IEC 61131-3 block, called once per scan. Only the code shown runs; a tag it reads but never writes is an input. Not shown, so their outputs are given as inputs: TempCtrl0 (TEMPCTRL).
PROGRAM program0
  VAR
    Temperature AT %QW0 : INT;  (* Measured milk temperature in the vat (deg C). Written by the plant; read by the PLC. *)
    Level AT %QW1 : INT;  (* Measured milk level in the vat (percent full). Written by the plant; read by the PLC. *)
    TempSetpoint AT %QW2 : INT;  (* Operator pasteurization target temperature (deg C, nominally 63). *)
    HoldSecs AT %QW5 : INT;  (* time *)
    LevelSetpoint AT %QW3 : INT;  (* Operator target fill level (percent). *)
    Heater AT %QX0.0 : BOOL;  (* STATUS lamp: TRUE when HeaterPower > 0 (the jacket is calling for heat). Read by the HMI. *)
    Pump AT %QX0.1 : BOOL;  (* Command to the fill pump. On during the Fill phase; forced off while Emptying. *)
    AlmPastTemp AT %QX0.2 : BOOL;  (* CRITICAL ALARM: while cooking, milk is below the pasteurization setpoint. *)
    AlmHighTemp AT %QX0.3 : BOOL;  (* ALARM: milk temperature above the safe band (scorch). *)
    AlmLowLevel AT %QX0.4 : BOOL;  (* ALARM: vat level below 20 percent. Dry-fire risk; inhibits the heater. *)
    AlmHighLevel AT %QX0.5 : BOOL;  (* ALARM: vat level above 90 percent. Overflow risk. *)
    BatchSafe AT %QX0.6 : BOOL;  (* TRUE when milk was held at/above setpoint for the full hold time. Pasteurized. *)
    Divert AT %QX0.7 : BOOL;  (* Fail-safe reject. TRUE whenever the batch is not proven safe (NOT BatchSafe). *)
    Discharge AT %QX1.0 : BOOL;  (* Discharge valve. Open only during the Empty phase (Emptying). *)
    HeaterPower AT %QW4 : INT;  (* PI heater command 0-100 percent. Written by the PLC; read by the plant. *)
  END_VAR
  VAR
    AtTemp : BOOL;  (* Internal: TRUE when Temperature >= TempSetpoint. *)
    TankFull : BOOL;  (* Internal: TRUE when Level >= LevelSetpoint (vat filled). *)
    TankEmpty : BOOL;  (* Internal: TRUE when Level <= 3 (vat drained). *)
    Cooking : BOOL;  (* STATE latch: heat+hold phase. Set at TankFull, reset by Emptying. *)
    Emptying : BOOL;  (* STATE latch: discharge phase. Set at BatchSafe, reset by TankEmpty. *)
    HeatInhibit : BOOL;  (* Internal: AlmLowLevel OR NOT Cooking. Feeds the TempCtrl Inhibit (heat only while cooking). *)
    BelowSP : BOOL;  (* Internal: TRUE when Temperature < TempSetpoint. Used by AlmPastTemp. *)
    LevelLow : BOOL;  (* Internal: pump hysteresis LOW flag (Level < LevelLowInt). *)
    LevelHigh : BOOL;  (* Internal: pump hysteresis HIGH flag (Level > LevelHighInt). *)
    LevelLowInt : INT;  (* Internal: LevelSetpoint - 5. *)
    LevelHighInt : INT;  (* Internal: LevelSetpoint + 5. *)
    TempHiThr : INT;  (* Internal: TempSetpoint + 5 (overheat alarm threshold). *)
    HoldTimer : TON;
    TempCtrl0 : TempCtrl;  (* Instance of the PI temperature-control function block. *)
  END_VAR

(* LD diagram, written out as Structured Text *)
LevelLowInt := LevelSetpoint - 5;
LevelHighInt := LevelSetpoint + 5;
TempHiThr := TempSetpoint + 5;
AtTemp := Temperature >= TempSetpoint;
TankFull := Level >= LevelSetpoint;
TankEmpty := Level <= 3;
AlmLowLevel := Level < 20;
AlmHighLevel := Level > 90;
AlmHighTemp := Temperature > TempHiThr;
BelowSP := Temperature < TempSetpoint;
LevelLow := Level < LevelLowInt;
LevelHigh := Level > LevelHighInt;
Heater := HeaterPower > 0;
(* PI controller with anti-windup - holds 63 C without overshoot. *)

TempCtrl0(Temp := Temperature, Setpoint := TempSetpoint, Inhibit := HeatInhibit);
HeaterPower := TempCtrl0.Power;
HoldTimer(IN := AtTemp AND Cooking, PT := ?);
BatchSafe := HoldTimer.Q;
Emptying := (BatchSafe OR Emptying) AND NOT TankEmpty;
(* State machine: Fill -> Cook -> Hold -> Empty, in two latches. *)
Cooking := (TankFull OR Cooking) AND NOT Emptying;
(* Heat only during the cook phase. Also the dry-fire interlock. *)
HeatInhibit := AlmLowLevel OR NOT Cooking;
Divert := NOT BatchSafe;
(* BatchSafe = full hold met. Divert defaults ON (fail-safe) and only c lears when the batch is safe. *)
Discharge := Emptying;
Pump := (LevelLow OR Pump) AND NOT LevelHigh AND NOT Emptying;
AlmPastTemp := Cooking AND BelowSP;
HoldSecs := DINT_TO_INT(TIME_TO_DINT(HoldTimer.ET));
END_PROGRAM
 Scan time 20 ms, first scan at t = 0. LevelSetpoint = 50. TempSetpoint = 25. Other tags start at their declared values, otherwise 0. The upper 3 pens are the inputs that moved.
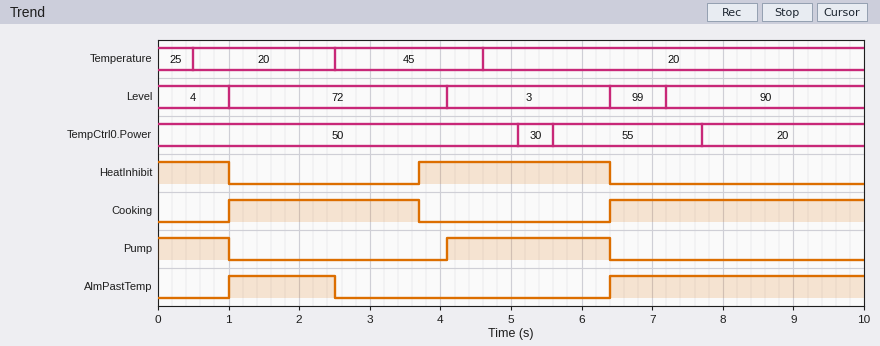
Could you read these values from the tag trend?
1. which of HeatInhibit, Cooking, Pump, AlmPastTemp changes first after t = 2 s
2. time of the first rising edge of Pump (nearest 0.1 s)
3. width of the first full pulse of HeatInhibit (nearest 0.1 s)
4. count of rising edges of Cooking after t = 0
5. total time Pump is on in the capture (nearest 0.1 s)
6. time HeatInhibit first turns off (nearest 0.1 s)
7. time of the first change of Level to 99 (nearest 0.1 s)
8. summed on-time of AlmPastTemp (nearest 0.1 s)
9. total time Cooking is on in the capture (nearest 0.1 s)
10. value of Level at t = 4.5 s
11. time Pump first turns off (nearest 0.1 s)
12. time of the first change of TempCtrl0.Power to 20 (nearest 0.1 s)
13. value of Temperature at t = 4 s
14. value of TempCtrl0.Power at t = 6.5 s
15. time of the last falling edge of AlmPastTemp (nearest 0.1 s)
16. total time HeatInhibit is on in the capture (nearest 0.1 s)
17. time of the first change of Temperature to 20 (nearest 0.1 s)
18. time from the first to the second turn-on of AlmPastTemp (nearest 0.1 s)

AlmPastTemp
4.1 s
2.7 s
2
3.3 s
1.0 s
6.4 s
5.1 s
6.3 s
3
1.0 s
7.7 s
45
55
2.5 s
3.7 s
0.5 s
5.4 s
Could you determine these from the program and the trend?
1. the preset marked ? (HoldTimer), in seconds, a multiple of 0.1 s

1.2 s
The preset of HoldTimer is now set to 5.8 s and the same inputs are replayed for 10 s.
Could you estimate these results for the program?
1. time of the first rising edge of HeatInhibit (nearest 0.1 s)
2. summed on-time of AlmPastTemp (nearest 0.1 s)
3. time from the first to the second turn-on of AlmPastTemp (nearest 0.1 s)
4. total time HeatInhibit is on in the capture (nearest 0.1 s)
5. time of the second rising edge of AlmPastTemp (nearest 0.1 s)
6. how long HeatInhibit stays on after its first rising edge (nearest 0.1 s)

4.1 s
6.9 s
3.6 s
3.3 s
4.6 s
2.3 s
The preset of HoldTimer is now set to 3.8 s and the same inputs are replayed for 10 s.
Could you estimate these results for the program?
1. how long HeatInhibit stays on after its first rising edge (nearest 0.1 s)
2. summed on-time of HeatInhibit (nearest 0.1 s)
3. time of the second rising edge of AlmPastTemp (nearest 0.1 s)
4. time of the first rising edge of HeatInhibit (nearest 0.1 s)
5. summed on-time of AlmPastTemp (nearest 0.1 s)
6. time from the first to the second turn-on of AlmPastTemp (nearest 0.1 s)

2.3 s
3.3 s
4.6 s
4.1 s
6.9 s
3.6 s
